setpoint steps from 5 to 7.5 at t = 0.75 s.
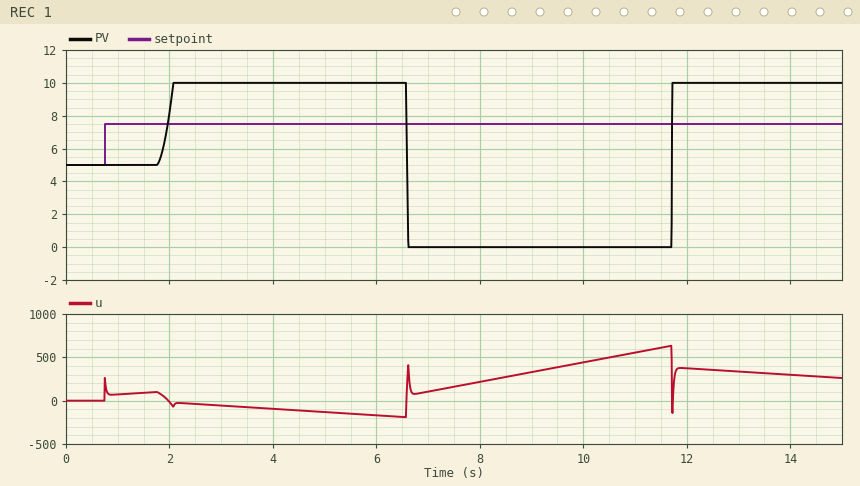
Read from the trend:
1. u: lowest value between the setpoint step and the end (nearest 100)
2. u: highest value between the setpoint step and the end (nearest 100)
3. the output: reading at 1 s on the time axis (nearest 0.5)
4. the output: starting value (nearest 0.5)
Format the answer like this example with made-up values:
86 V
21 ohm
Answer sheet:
-200
600
5.0
5.0
